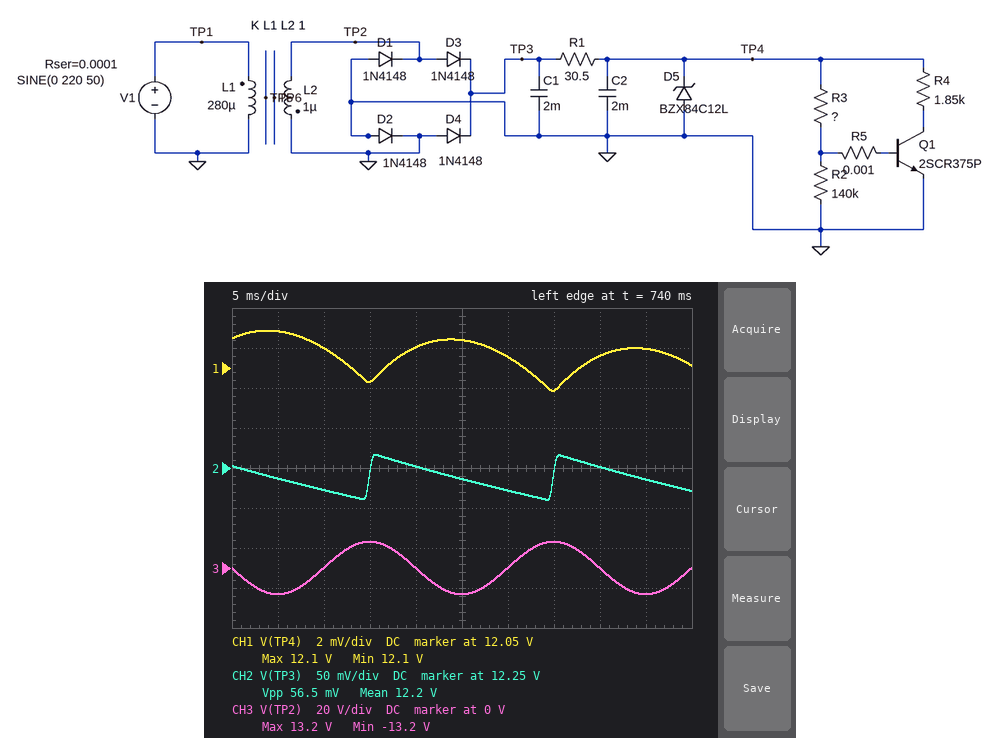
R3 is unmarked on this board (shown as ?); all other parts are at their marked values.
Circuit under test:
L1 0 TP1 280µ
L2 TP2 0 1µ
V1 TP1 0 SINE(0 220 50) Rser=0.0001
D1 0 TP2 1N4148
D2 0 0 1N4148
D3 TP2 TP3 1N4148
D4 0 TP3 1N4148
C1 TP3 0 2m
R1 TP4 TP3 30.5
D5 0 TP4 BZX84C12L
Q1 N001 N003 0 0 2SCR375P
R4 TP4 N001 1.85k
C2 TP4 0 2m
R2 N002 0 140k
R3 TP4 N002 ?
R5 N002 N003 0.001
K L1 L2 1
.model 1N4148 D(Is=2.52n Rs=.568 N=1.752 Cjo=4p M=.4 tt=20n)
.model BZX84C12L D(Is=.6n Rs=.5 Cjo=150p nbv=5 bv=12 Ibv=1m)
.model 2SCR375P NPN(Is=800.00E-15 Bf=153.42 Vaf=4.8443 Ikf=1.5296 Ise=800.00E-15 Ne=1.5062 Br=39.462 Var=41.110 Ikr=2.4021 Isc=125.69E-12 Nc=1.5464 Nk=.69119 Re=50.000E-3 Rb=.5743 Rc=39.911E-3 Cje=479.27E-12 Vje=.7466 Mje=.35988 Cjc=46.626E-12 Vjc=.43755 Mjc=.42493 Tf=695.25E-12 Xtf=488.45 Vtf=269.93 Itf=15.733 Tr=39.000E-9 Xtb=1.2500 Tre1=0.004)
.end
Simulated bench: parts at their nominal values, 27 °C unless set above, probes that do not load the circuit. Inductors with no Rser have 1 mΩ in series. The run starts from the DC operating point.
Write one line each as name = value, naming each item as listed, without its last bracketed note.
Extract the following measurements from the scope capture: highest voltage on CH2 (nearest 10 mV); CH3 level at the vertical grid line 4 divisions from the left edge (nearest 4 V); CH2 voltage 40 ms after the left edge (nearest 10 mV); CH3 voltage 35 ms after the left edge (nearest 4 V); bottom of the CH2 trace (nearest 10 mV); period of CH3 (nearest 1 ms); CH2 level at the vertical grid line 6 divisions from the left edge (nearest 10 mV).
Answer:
highest voltage on CH2 = 12.27 V
CH3 level at the vertical grid line 4 divisions from the left edge = 0 V
CH2 voltage 40 ms after the left edge = 12.25 V
CH3 voltage 35 ms after the left edge = 12 V
bottom of the CH2 trace = 12.21 V
period of CH3 = 20 ms
CH2 level at the vertical grid line 6 divisions from the left edge = 12.22 V
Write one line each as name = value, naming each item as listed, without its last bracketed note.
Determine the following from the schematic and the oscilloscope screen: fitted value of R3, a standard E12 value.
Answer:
fitted value of R3, a standard E12 value = 470 kΩ
